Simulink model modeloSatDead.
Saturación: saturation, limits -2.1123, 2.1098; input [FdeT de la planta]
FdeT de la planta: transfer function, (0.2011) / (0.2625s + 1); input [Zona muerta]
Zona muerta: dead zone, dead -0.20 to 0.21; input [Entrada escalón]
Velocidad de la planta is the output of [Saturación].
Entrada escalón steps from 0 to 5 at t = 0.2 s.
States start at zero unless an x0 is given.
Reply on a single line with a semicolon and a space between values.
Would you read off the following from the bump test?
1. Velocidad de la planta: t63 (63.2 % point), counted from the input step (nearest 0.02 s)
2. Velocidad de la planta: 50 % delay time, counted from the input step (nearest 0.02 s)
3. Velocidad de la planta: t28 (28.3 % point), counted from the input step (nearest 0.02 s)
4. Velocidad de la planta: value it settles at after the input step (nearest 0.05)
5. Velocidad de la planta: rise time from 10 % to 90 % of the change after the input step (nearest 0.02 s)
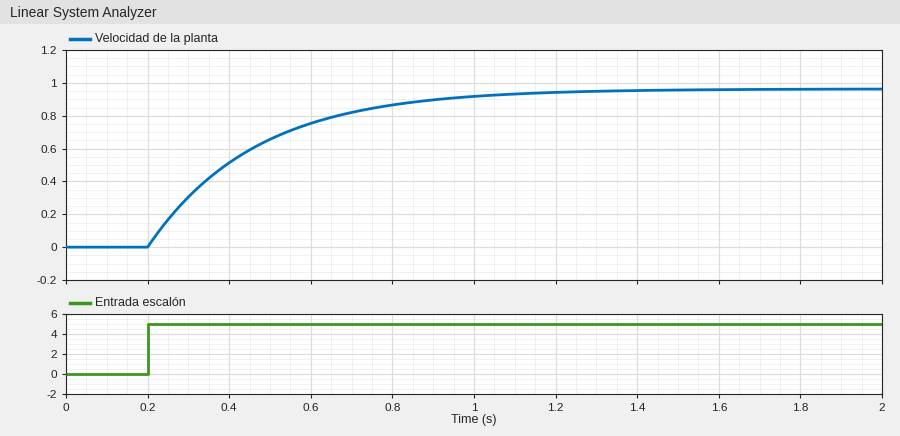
0.26 s; 0.18 s; 0.08 s; 0.95; 0.58 s
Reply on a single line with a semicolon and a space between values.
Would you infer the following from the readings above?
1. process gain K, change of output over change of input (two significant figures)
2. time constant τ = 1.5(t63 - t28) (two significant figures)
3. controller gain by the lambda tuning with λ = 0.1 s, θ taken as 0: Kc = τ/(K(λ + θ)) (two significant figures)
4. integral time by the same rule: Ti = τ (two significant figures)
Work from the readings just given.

0.19; 0.27 s; 14; 0.27 s
